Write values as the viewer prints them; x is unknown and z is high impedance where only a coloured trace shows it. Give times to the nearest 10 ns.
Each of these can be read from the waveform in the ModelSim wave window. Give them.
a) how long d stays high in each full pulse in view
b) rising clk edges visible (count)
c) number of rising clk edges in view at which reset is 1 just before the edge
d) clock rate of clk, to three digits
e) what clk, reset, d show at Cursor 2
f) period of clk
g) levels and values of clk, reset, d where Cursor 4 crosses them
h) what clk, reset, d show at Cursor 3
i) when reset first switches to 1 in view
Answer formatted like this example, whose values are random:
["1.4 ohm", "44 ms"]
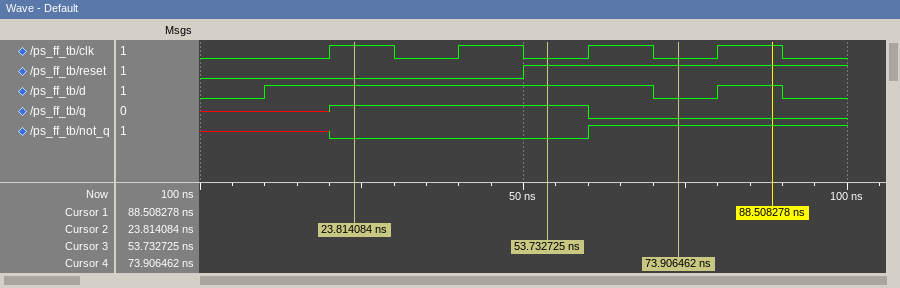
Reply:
["60 ns, 10 ns", "4", "2", "50.0 MHz", "clk=1, reset=0, d=1", "20 ns", "clk=0, reset=1, d=0", "clk=0, reset=1, d=1", "50 ns"]
